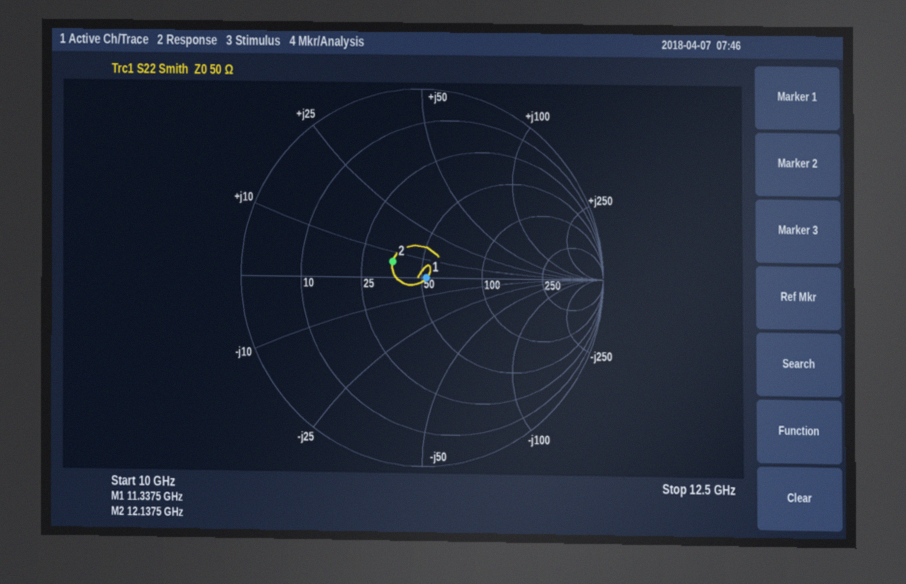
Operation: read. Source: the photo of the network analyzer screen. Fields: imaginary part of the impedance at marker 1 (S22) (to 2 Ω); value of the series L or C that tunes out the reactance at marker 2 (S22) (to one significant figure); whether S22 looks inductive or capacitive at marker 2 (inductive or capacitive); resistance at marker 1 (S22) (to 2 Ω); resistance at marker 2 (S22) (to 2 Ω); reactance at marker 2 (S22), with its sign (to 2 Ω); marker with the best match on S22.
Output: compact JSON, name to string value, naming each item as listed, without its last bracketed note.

{"imaginary part of the impedance at marker 1 (S22)": "0 Ω", "value of the series L or C that tunes out the reactance at marker 2 (S22)": "2 pF", "whether S22 looks inductive or capacitive at marker 2": "inductive", "resistance at marker 1 (S22)": "52 Ω", "resistance at marker 2 (S22)": "36 Ω", "reactance at marker 2 (S22), with its sign": "+6 Ω", "marker with the best match on S22": "marker 1"}
